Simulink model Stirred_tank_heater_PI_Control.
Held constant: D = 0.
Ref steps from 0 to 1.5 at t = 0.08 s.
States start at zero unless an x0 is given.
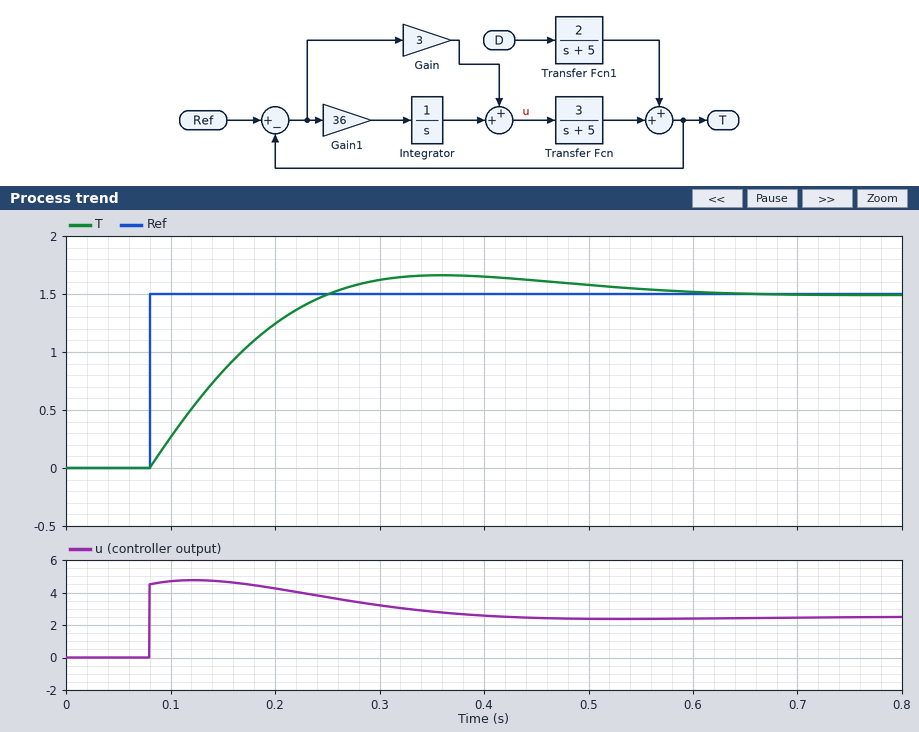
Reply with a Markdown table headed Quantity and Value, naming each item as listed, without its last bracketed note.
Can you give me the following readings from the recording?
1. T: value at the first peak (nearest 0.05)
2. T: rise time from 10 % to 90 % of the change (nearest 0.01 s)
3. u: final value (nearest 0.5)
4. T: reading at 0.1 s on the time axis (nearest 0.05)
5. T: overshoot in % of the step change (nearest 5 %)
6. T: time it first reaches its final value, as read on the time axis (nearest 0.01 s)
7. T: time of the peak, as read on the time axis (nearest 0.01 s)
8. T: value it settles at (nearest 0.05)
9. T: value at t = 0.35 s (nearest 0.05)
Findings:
| Quantity | Value |
|---|---|
| T: value at the first peak | 1.65 |
| T: rise time from 10 % to 90 % of the change | 0.13 s |
| u: final value | 2.5 |
| T: reading at 0.1 s on the time axis | 0.25 |
| T: overshoot in % of the step change | 10 % |
| T: time it first reaches its final value, as read on the time axis | 0.25 s |
| T: time of the peak, as read on the time axis | 0.36 s |
| T: value it settles at | 1.50 |
| T: value at t = 0.35 s | 1.65 |
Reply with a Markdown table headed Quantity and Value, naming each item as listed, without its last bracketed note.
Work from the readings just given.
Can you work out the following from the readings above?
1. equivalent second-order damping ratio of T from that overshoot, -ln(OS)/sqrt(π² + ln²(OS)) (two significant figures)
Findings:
| Quantity | Value |
|---|---|
| equivalent second-order damping ratio of T from that overshoot, -ln(OS)/sqrt(π² + ln²(OS)) | 0.59 |
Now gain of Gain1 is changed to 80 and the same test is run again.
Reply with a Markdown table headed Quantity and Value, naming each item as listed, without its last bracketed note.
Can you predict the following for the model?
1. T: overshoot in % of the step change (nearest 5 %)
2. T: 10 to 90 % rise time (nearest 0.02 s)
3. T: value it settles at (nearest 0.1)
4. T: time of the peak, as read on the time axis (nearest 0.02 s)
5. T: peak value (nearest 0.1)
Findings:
| Quantity | Value |
|---|---|
| T: overshoot in % of the step change | 25 % |
| T: 10 to 90 % rise time | 0.08 s |
| T: value it settles at | 1.5 |
| T: time of the peak, as read on the time axis | 0.26 s |
| T: peak value | 1.9 |
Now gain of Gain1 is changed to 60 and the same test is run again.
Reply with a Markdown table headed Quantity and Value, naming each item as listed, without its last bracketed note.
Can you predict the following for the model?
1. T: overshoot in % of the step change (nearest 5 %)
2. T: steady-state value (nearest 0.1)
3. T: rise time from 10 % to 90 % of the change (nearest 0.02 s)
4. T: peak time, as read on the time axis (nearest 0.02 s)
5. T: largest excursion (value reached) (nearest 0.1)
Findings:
| Quantity | Value |
|---|---|
| T: overshoot in % of the step change | 20 % |
| T: steady-state value | 1.5 |
| T: rise time from 10 % to 90 % of the change | 0.10 s |
| T: peak time, as read on the time axis | 0.30 s |
| T: largest excursion (value reached) | 1.8 |
